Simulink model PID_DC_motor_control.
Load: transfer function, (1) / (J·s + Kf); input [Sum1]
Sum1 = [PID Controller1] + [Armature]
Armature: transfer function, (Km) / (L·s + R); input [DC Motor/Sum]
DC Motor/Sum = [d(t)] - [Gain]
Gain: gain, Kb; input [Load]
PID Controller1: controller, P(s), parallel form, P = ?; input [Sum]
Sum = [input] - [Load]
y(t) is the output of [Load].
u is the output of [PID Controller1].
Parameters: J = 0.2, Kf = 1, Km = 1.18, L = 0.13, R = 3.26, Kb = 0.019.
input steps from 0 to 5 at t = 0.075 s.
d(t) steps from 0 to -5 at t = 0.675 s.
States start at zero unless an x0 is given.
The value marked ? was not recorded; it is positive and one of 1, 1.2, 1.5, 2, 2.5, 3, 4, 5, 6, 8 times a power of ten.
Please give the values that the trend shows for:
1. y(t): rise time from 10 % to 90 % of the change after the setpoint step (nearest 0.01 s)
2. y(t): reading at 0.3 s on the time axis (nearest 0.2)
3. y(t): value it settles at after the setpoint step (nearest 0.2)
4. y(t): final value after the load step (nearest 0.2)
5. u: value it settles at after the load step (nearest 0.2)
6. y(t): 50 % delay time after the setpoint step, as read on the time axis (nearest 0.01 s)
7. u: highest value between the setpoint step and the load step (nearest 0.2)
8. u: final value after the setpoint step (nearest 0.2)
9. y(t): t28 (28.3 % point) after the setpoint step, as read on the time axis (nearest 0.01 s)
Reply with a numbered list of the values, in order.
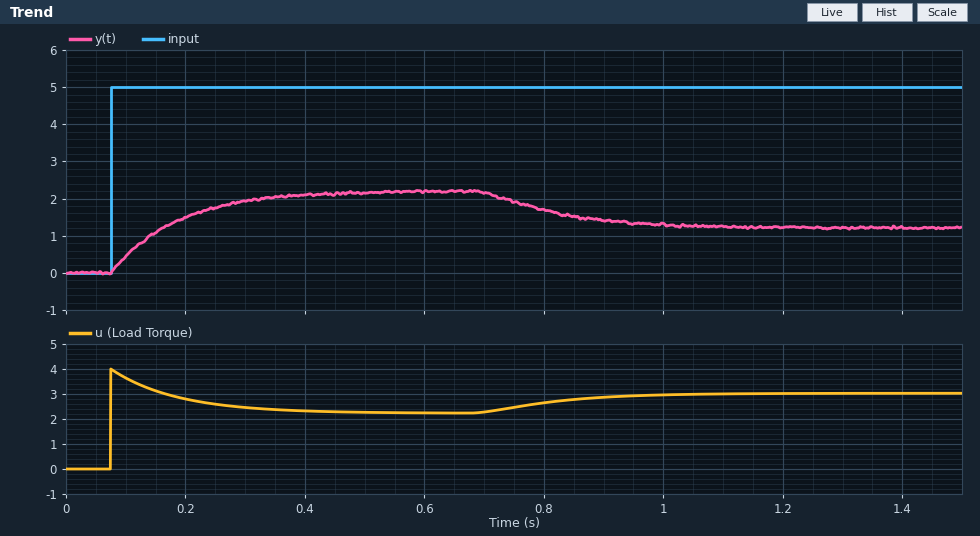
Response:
1. 0.24 s
2. 2.0
3. 2.2
4. 1.2
5. 3.0
6. 0.15 s
7. 4.0
8. 2.2
9. 0.11 s
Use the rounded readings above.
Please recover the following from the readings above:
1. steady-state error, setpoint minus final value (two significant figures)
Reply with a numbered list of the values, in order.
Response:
1. 2.8
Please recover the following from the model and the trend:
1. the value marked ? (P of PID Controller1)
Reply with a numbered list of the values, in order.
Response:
1. 0.8
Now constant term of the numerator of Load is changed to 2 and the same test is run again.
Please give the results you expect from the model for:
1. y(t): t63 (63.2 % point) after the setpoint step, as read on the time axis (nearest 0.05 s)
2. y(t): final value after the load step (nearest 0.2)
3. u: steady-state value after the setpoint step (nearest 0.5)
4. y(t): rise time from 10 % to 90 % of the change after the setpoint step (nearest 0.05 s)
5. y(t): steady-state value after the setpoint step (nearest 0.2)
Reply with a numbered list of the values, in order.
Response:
1. 0.15 s
2. 1.6
3. 1.5
4. 0.15 s
5. 3.0
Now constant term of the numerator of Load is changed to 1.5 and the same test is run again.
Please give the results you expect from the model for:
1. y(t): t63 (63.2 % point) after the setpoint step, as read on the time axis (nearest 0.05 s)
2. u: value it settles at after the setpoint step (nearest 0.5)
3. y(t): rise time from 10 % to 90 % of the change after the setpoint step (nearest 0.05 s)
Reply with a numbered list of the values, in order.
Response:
1. 0.15 s
2. 2.0
3. 0.20 s
